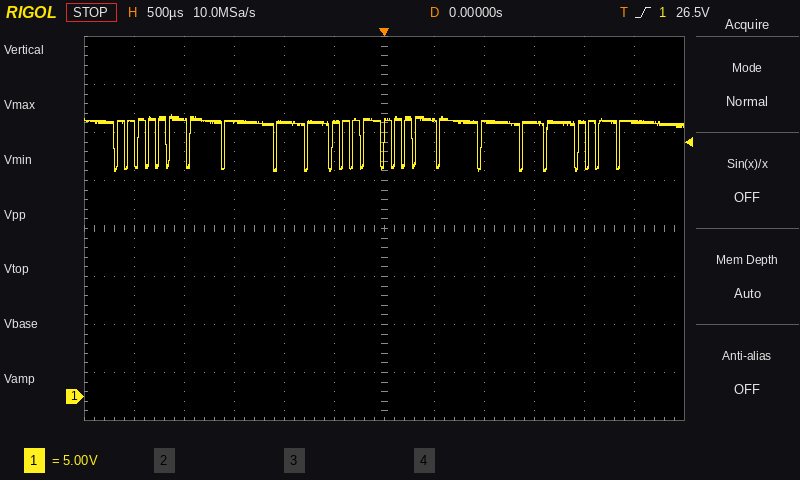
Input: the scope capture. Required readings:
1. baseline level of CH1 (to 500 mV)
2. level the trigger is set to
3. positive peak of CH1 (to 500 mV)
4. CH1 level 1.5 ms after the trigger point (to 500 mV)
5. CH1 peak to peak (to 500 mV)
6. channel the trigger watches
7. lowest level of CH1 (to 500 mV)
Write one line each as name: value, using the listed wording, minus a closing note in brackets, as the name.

baseline level of CH1: 28.5 V
level the trigger is set to: 26.5 V
positive peak of CH1: 29.5 V
CH1 level 1.5 ms after the trigger point: 28.5 V
CH1 peak to peak: 6.0 V
channel the trigger watches: CH1
lowest level of CH1: 23.5 V
